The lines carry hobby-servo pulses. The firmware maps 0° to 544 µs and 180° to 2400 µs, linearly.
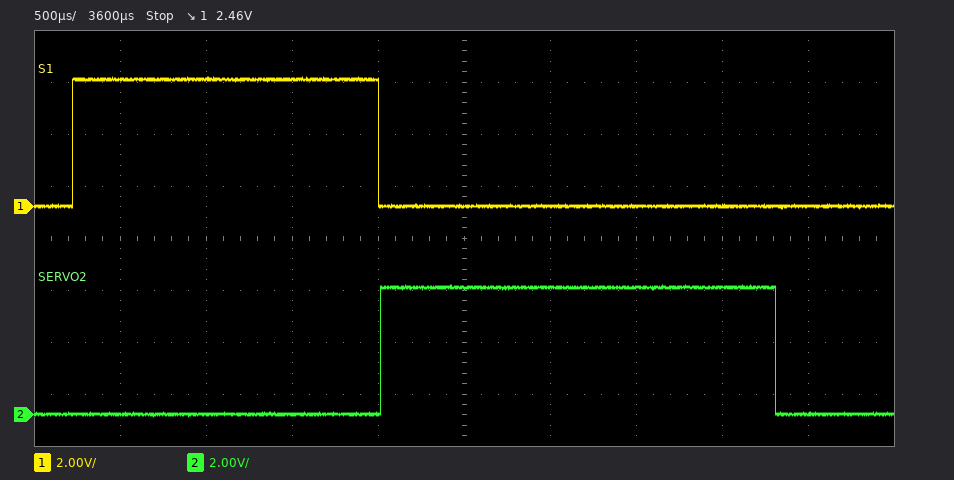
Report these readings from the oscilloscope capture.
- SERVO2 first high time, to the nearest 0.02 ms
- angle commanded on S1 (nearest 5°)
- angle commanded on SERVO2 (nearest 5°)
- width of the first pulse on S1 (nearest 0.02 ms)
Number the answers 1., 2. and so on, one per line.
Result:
1. 2.30 ms
2. 120°
3. 170°
4. 1.78 ms
